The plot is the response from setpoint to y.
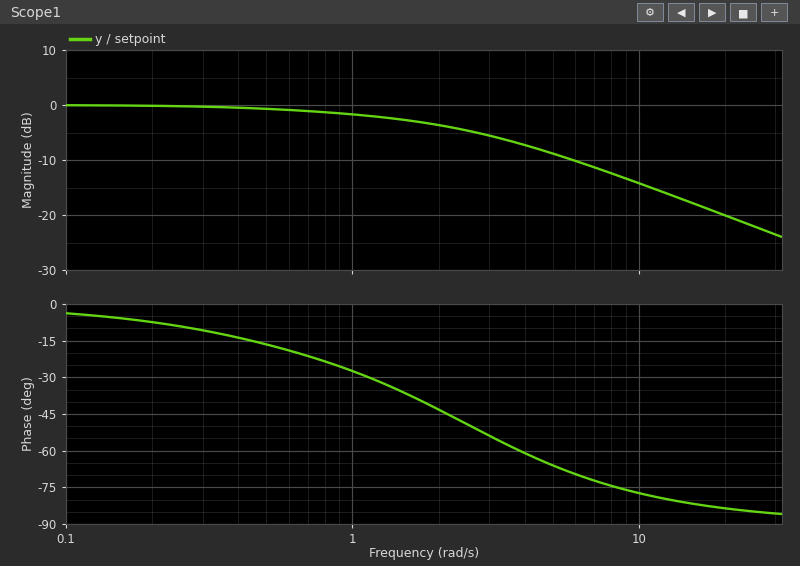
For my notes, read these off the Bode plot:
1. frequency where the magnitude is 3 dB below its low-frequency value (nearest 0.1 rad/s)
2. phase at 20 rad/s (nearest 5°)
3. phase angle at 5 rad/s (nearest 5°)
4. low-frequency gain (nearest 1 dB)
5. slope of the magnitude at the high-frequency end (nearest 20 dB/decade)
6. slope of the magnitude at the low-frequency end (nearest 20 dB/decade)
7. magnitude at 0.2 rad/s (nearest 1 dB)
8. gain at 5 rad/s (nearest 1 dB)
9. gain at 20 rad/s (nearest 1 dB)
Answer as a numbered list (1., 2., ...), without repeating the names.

1. 1.7 rad/s
2. -85°
3. -65°
4. 0 dB
5. -20 dB/decade
6. 0 dB/decade
7. 0 dB
8. -9 dB
9. -20 dB
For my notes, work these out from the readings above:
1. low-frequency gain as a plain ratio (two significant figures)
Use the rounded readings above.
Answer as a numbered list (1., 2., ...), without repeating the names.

1. 1.0
